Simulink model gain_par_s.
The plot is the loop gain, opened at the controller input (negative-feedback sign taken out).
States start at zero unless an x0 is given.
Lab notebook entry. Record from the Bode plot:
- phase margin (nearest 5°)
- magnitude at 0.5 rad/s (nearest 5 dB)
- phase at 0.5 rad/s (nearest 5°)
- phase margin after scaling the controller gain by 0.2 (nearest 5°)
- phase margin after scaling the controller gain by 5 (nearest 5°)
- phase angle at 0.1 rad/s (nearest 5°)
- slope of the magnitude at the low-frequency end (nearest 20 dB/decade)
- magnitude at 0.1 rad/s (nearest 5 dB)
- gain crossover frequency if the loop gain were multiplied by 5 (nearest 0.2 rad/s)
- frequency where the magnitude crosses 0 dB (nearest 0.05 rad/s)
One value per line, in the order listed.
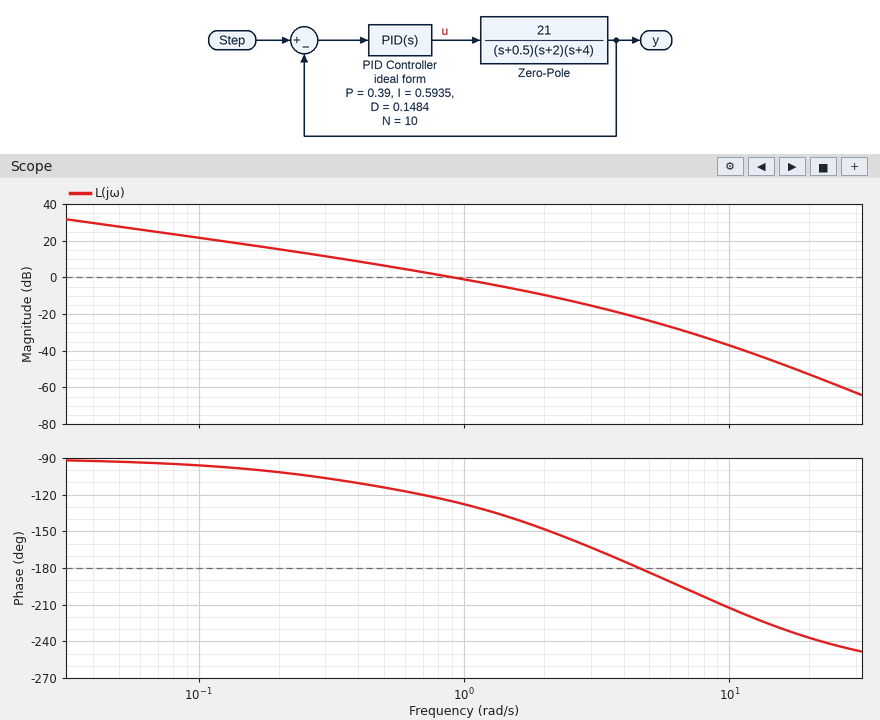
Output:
55°
5 dB
-115°
75°
20°
-95°
-20 dB/decade
20 dB
2.8 rad/s
0.90 rad/s
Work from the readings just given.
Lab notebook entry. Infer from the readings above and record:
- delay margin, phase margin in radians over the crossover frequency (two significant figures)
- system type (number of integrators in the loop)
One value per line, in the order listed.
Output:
1.1 s
1
